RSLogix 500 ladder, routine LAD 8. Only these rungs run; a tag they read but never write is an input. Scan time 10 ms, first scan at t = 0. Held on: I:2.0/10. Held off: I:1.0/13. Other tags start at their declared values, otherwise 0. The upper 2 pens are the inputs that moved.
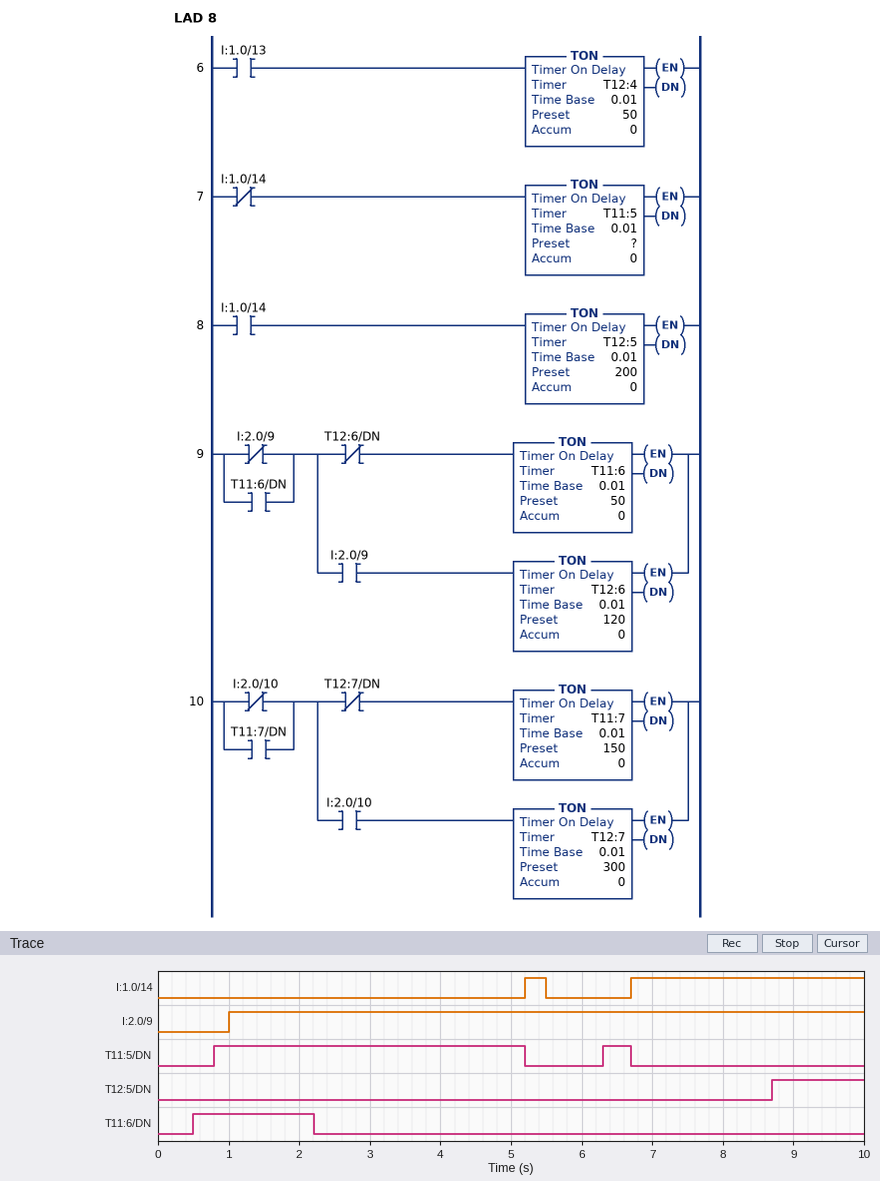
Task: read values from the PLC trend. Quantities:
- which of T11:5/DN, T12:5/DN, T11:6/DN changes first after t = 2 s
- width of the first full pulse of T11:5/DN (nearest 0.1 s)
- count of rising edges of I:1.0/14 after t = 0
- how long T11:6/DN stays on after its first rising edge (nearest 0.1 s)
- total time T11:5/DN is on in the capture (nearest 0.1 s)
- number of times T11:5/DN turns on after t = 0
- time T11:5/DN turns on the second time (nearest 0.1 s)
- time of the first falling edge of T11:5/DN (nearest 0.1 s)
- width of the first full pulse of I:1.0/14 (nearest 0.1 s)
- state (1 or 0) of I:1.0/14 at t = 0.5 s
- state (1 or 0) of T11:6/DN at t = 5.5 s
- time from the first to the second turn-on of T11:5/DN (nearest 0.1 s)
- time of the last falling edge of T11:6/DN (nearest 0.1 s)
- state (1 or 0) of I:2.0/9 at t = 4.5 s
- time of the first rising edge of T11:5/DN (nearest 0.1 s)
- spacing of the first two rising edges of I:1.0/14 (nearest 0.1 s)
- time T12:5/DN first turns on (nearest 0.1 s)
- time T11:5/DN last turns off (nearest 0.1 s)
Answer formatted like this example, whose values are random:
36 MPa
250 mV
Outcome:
T11:6/DN
4.4 s
2
1.7 s
4.8 s
2
6.3 s
5.2 s
0.3 s
0
0
5.5 s
2.2 s
1
0.8 s
1.5 s
8.7 s
6.7 s
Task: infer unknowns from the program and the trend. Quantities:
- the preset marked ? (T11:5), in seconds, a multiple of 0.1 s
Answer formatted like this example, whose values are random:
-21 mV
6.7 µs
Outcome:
0.8 s
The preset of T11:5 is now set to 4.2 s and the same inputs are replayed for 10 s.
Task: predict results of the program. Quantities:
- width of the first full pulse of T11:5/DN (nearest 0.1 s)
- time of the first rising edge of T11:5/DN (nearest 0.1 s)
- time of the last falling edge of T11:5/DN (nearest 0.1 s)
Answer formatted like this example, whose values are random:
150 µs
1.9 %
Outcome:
1.0 s
4.2 s
5.2 s
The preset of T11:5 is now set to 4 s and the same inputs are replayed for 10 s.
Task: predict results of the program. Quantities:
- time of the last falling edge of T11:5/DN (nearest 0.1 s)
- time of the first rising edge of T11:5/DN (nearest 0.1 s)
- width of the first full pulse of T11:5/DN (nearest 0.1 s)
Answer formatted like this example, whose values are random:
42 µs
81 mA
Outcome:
5.2 s
4.0 s
1.2 s
